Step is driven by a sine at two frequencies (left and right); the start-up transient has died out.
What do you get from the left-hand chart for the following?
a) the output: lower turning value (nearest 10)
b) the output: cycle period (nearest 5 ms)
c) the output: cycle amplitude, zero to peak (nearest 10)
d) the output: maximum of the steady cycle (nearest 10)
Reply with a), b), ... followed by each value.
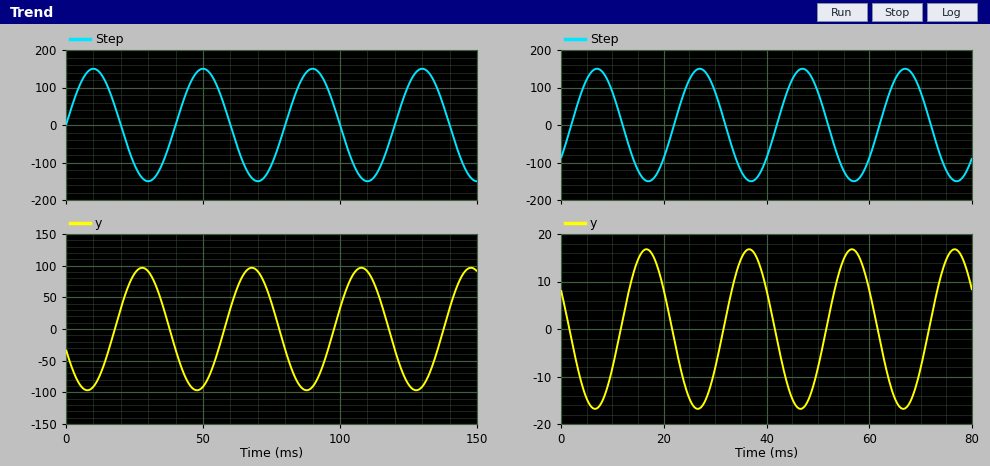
a) -100
b) 40 ms
c) 100
d) 100
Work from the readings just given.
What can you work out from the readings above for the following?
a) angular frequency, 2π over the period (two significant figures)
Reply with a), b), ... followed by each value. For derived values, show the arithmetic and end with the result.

a) 2π / 40 = 0.16 rad/ms
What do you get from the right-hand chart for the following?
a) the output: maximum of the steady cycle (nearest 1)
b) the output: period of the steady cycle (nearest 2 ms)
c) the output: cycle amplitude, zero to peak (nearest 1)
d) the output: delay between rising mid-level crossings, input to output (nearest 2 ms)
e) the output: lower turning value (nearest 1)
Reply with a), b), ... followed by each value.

a) 17
b) 20 ms
c) 17
d) 10 ms
e) -17
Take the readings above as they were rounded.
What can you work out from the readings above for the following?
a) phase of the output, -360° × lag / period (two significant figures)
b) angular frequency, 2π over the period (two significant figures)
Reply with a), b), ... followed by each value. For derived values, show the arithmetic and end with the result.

a) -360 × 10 / 20 = -180°
b) 2π / 20 = 0.31 rad/ms
